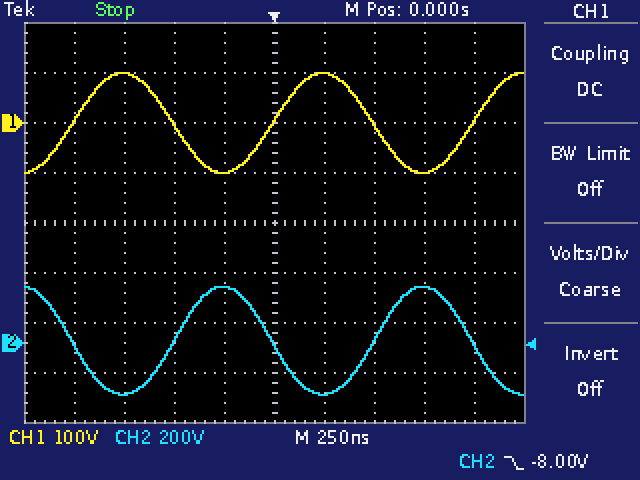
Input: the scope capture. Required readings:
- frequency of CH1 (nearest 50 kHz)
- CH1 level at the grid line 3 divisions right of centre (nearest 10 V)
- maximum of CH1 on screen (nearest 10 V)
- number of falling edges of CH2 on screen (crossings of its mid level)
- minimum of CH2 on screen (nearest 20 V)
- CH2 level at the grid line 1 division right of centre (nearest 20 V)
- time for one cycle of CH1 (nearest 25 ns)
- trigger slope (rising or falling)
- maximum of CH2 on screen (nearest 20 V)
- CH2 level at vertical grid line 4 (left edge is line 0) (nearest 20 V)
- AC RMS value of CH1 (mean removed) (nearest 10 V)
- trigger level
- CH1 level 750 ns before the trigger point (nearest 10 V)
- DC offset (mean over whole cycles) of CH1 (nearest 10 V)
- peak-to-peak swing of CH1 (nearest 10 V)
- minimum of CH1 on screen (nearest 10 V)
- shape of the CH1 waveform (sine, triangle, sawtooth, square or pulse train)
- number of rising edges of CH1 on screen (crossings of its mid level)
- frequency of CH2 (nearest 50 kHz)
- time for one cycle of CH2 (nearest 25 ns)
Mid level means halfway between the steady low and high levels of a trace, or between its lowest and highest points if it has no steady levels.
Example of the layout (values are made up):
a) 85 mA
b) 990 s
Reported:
a) 1.00 MHz
b) -100 V
c) 100 V
d) 3
e) -200 V
f) -200 V
g) 1.000 µs
h) falling
i) 220 V
j) 220 V
k) 70 V
l) -8.00 V
m) 100 V
n) 0 V
o) 200 V
p) -100 V
q) sine
r) 3
s) 1.00 MHz
t) 1.000 µs
